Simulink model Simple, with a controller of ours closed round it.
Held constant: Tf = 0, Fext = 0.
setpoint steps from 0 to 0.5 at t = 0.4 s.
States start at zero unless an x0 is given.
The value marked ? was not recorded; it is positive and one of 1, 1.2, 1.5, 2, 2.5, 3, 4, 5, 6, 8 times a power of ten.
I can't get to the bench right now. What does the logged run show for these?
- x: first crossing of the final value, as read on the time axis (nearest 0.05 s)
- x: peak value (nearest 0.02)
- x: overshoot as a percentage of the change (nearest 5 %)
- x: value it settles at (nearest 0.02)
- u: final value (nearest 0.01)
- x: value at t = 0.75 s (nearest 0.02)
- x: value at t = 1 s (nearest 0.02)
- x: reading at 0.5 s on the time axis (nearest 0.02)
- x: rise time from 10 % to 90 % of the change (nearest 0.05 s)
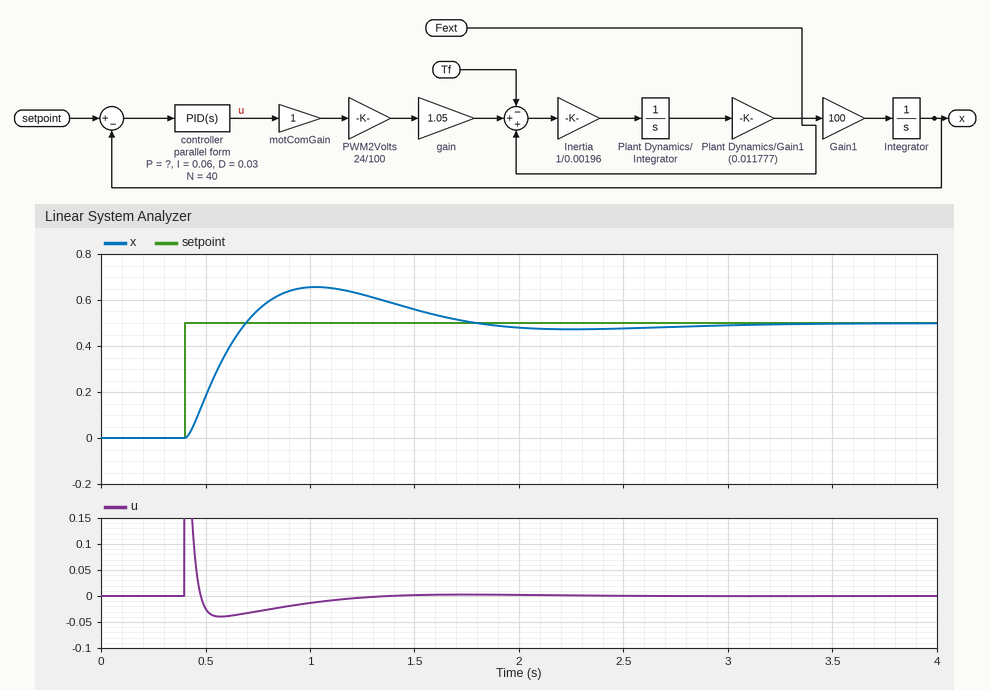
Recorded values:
0.70 s
0.66
30 %
0.50
0.00
0.56
0.66
0.18
0.20 s
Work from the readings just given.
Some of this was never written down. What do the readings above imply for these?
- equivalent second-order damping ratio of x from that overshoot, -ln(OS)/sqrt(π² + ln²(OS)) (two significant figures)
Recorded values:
0.36
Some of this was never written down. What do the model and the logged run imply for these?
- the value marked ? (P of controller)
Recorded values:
0.08
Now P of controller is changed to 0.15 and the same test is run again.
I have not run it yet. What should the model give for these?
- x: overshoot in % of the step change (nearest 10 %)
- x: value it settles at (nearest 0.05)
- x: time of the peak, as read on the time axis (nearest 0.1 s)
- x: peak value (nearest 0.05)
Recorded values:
40 %
0.50
0.9 s
0.70
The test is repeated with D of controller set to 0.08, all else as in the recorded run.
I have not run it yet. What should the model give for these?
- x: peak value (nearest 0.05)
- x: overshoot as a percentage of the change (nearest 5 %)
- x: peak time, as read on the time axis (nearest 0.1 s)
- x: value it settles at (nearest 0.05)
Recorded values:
0.55
10 %
0.7 s
0.50
